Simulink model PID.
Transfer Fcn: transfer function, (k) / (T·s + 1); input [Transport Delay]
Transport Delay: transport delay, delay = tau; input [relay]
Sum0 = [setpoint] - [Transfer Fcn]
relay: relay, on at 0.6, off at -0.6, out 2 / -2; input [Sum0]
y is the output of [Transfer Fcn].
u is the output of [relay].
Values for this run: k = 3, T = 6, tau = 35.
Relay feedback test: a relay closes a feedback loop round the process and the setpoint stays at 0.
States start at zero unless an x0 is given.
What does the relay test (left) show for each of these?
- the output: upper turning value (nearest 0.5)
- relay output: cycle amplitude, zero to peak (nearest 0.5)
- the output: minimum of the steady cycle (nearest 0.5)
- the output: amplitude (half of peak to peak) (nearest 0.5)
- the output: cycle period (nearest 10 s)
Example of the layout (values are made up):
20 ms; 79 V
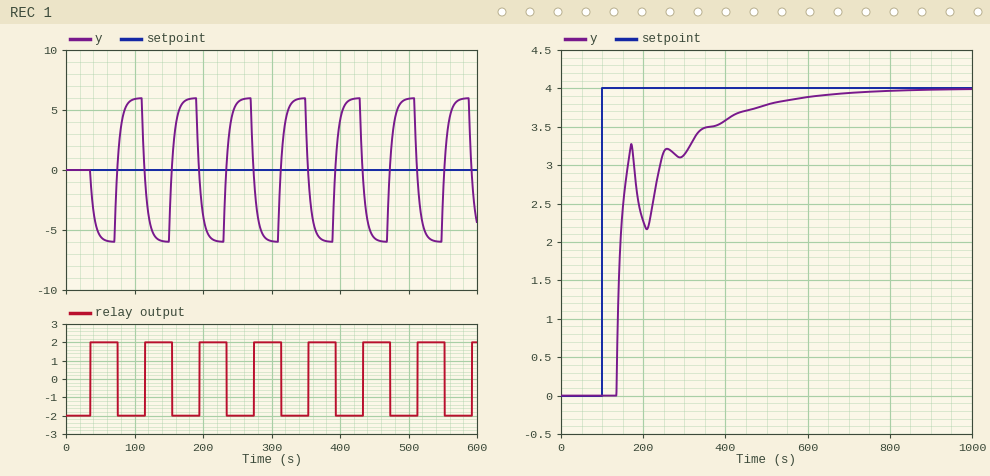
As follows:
6.0; 2.0; -6.0; 6.0; 80 s
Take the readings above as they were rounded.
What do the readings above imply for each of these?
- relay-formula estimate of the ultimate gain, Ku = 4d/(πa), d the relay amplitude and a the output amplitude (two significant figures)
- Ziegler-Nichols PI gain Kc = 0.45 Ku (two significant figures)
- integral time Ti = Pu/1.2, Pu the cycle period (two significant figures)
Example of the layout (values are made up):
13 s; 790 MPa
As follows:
0.42; 0.19; 67 s
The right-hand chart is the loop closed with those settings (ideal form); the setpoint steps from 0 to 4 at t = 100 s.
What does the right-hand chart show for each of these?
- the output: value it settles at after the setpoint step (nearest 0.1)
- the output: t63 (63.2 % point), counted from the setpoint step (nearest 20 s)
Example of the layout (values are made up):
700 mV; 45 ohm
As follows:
4.0; 60 s
